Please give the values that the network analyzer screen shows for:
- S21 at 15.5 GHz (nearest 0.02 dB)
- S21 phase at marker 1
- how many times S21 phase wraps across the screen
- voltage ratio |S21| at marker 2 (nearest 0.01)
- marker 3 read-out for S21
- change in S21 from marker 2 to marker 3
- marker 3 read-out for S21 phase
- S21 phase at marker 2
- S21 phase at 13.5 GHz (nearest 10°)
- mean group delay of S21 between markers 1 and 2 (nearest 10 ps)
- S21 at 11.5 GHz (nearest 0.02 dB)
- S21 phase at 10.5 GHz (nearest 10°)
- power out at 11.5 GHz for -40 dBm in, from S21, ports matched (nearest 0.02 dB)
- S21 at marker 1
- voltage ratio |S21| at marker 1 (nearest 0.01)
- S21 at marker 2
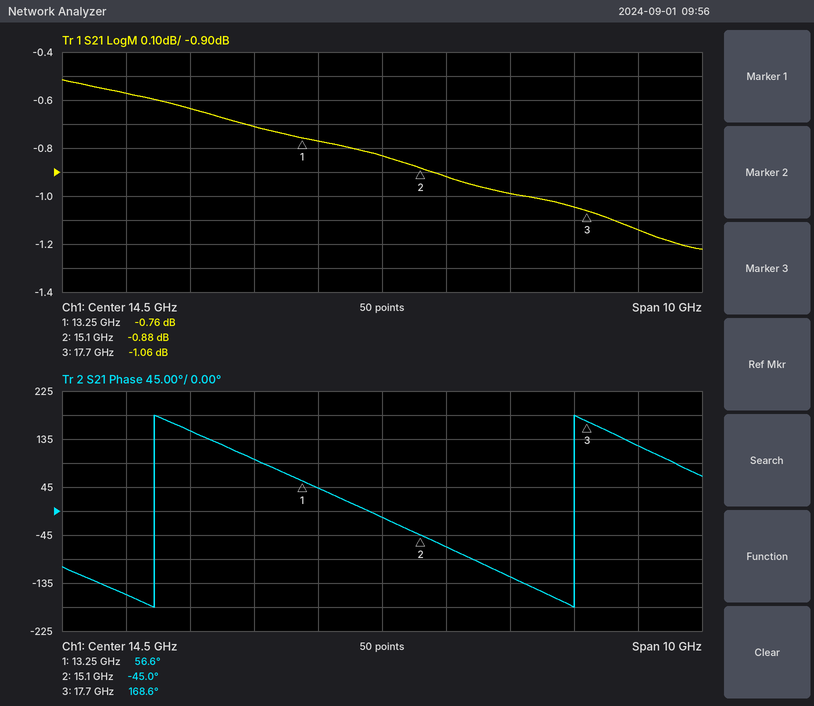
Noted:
-0.92 dB
56.6°
2
0.90
-1.06 dB
-0.18 dB
168.6°
-45.0°
40°
150 ps
-0.64 dB
-160°
-40.64 dBm
-0.76 dB
0.92
-0.88 dB
